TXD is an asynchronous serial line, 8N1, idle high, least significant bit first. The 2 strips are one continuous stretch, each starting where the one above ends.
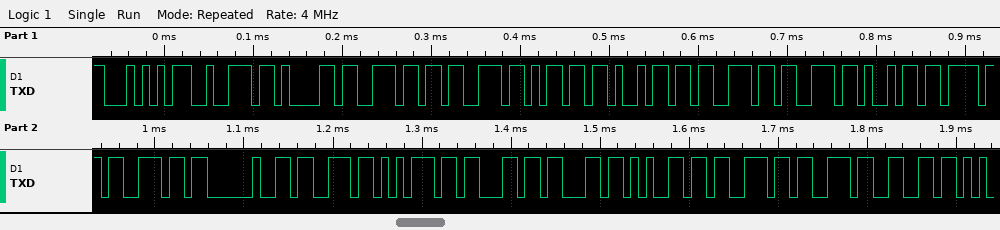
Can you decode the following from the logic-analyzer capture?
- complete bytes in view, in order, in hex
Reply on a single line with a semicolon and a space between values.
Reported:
54 72 61 6E 73 6D 69 73 73 69 6F 6E 20 73 75 63 63 65 73 73 66
